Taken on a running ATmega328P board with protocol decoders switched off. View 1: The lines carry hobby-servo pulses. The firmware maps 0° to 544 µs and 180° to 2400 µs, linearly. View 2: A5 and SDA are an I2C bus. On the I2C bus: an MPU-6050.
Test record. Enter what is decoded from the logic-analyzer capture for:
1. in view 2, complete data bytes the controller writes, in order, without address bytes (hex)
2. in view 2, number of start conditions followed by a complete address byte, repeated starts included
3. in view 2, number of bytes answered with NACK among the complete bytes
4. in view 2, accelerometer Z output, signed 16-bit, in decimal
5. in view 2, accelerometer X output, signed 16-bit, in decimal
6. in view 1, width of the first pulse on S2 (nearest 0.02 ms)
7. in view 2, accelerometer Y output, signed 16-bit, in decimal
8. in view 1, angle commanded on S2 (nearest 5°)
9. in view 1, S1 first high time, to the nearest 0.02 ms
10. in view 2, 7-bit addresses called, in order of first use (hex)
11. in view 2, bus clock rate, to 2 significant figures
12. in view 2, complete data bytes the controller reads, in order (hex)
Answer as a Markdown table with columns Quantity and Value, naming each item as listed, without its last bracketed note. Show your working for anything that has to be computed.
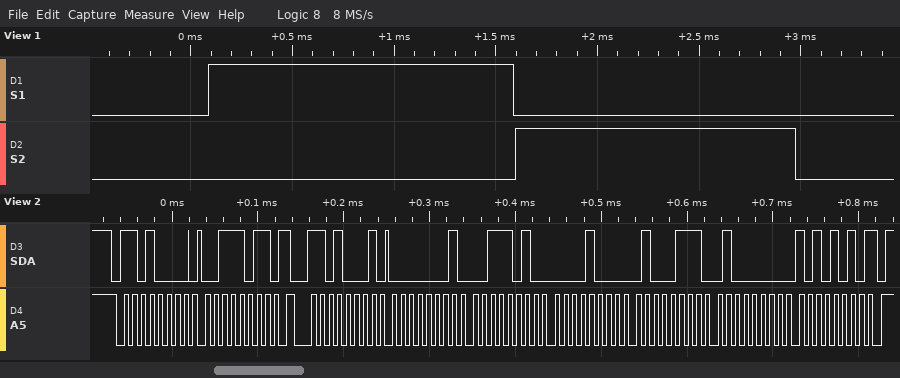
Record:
| Quantity | Value |
|---|---|
| in view 2, complete data bytes the controller writes, in order, without address bytes | 3B |
| in view 2, number of start conditions followed by a complete address byte, repeated starts included | 2 |
| in view 2, number of bytes answered with NACK among the complete bytes | 1 |
| in view 2, accelerometer Z output, signed 16-bit, in decimal | 0x40AA = 16554 |
| in view 2, accelerometer X output, signed 16-bit, in decimal | 0x013A = 314 |
| in view 1, width of the first pulse on S2 | 1.38 ms |
| in view 2, accelerometer Y output, signed 16-bit, in decimal | 0x0847 = 2119 |
| in view 1, angle commanded on S2 | 80° |
| in view 1, S1 first high time, to the nearest 0.02 ms | 1.50 ms |
| in view 2, 7-bit addresses called, in order of first use | 0x68 |
| in view 2, bus clock rate, to 2 significant figures | 100 kHz |
| in view 2, complete data bytes the controller reads, in order | 01 3A 08 47 40 AA |
